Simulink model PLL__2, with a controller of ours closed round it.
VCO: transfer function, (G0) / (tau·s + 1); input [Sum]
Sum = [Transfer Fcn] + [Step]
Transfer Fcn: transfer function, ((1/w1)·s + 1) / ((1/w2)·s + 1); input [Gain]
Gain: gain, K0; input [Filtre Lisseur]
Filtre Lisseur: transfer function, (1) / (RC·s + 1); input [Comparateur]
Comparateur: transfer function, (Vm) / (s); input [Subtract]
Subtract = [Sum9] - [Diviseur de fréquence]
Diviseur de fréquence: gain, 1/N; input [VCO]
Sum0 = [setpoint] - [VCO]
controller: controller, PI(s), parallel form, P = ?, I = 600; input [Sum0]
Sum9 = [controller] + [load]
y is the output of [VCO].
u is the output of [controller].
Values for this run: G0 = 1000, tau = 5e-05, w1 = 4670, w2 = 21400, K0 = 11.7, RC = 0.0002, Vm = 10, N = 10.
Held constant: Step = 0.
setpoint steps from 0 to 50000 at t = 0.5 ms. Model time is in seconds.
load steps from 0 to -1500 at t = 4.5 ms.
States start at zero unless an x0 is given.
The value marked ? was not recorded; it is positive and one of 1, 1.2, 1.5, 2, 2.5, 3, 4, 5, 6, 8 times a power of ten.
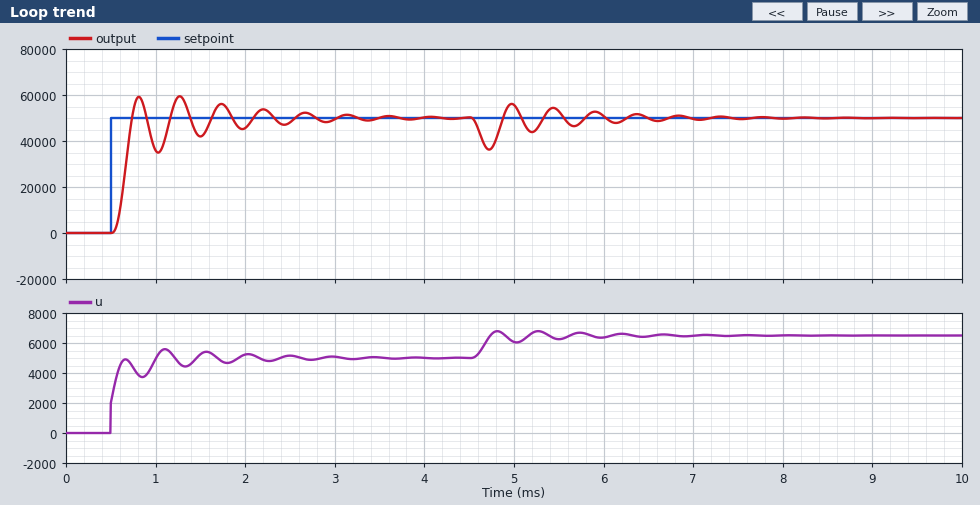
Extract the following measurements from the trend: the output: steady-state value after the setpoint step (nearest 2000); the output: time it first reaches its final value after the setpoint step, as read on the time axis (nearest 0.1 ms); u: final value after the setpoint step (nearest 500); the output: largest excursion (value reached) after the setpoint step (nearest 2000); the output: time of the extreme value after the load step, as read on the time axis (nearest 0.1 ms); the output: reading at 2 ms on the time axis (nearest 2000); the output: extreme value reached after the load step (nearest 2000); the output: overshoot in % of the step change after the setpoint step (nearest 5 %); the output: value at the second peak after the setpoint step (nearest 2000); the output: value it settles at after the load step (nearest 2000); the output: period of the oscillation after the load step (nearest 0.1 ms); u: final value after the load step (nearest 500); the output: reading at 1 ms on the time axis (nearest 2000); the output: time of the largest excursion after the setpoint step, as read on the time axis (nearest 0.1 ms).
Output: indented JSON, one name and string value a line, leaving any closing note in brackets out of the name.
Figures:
{
  "the output: steady-state value after the setpoint step": "50000",
  "the output: time it first reaches its final value after the setpoint step, as read on the time axis": "0.7 ms",
  "u: final value after the setpoint step": "5000",
  "the output: largest excursion (value reached) after the setpoint step": "60000",
  "the output: time of the extreme value after the load step, as read on the time axis": "4.7 ms",
  "the output: reading at 2 ms on the time axis": "46000",
  "the output: extreme value reached after the load step": "36000",
  "the output: overshoot in % of the step change after the setpoint step": "20 %",
  "the output: value at the second peak after the setpoint step": "60000",
  "the output: value it settles at after the load step": "50000",
  "the output: period of the oscillation after the load step": "0.5 ms",
  "u: final value after the load step": "6500",
  "the output: reading at 1 ms on the time axis": "36000",
  "the output: time of the largest excursion after the setpoint step, as read on the time axis": "1.3 ms"
}
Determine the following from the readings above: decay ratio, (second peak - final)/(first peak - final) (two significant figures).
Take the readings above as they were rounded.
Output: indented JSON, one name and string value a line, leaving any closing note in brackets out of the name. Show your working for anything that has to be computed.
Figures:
{
  "decay ratio, (second peak - final)/(first peak - final)": "(60000 - 50000) / (60000 - 50000) = 1.0"
}
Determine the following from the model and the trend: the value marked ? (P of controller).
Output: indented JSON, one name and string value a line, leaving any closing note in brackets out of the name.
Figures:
{
  "the value marked ?": "0.04"
}
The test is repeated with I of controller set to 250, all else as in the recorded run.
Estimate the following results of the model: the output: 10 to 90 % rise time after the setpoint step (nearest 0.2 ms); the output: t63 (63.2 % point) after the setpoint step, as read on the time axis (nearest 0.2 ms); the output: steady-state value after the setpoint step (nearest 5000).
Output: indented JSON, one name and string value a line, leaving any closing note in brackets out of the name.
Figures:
{
  "the output: 10 to 90 % rise time after the setpoint step": "1.0 ms",
  "the output: t63 (63.2 % point) after the setpoint step, as read on the time axis": "0.8 ms",
  "the output: steady-state value after the setpoint step": "50000"
}
